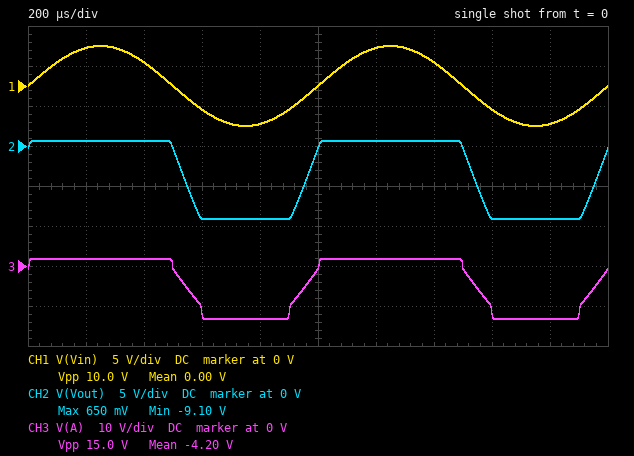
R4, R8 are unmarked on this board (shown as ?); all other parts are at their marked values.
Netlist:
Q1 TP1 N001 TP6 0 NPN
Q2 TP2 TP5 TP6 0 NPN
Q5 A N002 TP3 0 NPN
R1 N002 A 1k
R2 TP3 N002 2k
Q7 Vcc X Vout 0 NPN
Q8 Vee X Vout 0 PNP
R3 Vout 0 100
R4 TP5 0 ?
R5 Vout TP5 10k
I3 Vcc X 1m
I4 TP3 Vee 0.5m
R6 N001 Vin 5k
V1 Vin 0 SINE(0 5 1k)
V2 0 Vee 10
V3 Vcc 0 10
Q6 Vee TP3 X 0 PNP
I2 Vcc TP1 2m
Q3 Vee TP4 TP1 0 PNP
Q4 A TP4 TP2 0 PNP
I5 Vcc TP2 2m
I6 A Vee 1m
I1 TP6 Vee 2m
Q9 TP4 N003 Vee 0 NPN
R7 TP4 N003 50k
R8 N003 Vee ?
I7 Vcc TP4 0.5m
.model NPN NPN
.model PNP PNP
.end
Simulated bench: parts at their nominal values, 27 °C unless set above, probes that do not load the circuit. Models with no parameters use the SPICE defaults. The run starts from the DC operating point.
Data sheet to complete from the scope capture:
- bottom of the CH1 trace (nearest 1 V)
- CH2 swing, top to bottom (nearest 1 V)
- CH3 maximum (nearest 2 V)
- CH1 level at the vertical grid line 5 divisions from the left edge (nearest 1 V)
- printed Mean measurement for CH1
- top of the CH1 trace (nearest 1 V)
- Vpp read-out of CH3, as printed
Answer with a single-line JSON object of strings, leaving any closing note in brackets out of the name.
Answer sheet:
{"bottom of the CH1 trace": "-5 V", "CH2 swing, top to bottom": "10 V", "CH3 maximum": "2 V", "CH1 level at the vertical grid line 5 divisions from the left edge": "0 V", "printed Mean measurement for CH1": "0.00 V", "top of the CH1 trace": "5 V", "Vpp read-out of CH3, as printed": "15.0 V"}
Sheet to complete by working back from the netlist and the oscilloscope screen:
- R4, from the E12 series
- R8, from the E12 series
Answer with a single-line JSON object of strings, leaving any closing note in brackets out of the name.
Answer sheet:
{"R4, from the E12 series": "4.7 kΩ", "R8, from the E12 series": "3.9 kΩ"}
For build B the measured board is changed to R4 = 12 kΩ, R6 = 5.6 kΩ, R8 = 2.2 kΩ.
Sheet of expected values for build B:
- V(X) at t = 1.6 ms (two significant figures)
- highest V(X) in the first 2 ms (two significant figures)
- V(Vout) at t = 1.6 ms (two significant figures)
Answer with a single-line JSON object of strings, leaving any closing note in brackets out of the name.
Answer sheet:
{"V(X) at t = 1.6 ms": "-6.4 V", "highest V(X) in the first 2 ms": "8.8 V", "V(Vout) at t = 1.6 ms": "-5.5 V"}
